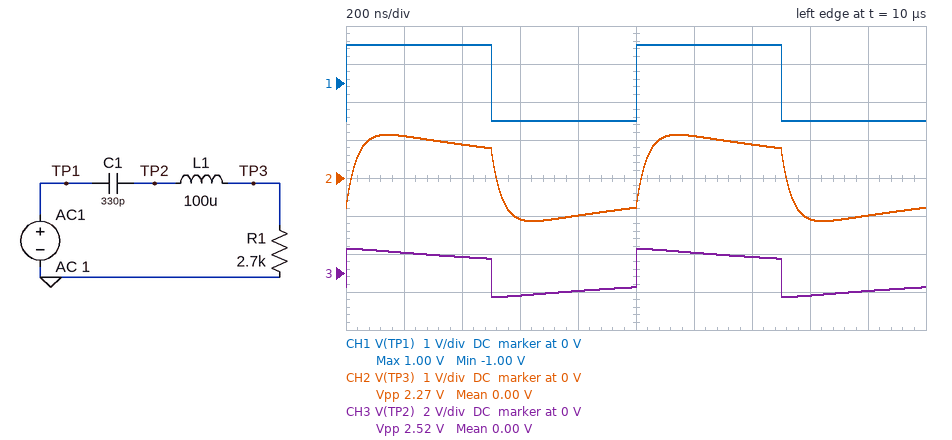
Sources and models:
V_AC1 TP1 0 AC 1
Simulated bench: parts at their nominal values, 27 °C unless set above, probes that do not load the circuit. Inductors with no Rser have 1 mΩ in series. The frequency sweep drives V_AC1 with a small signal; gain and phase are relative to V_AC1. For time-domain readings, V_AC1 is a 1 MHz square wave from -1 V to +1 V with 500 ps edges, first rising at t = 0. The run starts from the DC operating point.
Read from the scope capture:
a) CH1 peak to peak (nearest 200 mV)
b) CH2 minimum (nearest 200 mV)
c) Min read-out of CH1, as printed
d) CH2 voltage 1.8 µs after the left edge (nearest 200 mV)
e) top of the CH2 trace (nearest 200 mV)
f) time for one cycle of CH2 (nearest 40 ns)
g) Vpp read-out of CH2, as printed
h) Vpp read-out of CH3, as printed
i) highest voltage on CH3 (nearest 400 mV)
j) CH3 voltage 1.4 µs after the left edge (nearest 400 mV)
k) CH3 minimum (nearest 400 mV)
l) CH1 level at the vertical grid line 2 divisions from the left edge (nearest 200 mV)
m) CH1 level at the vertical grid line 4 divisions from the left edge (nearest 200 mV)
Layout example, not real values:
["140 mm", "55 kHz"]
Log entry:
["2.0 V", "-1.2 V", "-1.00 V", "-1.0 V", "1.2 V", "1.00 µs", "2.27 V", "2.52 V", "1.2 V", "800 mV", "-1.2 V", "1.0 V", "-1.0 V"]
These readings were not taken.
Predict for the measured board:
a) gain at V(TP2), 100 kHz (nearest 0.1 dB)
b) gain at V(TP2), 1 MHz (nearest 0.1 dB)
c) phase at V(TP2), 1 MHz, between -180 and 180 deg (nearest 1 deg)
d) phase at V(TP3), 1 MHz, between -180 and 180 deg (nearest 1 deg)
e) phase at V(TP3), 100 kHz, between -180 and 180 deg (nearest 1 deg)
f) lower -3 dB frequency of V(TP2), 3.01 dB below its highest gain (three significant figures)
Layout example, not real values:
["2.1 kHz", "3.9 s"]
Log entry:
["-6.1 dB", "0.2 dB", "10 deg", "-3 deg", "60 deg", "182 kHz"]
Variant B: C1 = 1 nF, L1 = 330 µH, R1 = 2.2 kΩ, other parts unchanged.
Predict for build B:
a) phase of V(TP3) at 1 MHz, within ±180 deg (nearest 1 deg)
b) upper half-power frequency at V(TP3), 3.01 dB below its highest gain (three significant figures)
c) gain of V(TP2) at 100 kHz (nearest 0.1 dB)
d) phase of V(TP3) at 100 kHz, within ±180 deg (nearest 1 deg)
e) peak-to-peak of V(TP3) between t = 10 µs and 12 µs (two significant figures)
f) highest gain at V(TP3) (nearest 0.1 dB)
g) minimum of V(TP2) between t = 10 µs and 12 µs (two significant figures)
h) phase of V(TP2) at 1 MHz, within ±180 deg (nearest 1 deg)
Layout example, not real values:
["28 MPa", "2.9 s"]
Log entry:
["-41 deg", "1.13 MHz", "-1.4 dB", "32 deg", "1.9 V", "0 dB", "-1.1 V", "2 deg"]
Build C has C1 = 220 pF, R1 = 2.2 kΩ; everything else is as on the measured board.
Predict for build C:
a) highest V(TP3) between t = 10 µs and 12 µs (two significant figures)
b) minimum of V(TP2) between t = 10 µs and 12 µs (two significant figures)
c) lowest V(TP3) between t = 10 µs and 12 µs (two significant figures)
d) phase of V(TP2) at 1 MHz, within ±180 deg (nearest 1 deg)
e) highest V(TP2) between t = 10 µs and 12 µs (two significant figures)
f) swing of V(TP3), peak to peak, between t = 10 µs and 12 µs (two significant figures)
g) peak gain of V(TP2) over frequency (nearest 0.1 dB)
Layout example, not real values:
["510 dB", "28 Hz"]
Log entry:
["1.2 V", "-1.5 V", "-1.2 V", "18 deg", "1.5 V", "2.5 V", "0.6 dB"]
